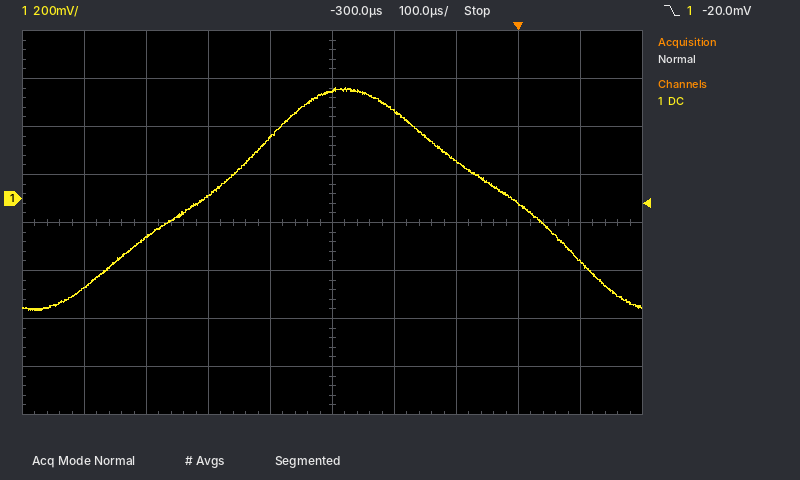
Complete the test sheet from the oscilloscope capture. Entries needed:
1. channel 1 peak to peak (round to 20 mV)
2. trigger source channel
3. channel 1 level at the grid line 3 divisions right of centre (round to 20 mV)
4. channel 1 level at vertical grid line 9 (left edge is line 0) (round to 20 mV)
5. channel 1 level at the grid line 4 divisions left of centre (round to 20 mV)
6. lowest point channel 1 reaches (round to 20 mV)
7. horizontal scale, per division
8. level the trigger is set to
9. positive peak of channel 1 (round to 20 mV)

920 mV
channel 1
-20 mV
-260 mV
-380 mV
-460 mV
100 µs
-20.0 mV
460 mV
